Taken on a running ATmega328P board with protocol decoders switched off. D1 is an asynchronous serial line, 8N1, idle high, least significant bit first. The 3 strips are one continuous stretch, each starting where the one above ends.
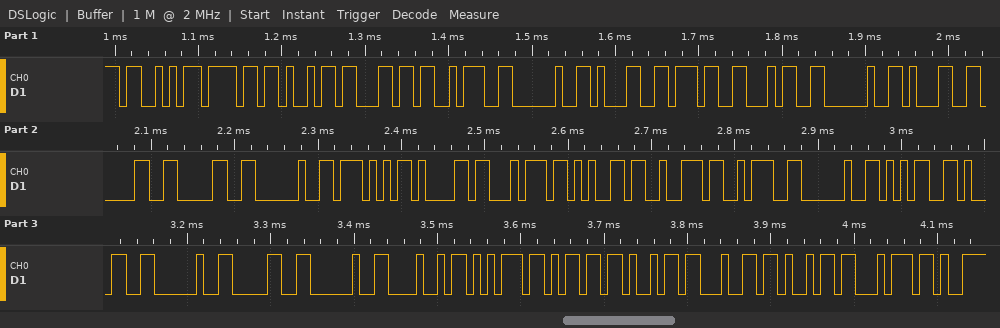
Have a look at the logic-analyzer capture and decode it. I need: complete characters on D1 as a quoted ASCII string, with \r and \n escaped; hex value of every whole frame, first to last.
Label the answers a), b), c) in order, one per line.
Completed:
a) "Soil: 174 100 Water: 51 0 Humidit"
b) 0x53 0x6F 0x69 0x6C 0x3A 0x20 0x31 0x37 0x34 0x20 0x31 0x30 0x30 0x20 0x57 0x61 0x74 0x65 0x72 0x3A 0x20 0x35 0x31 0x20 0x30 0x20 0x48 0x75 0x6D 0x69 0x64 0x69 0x74
